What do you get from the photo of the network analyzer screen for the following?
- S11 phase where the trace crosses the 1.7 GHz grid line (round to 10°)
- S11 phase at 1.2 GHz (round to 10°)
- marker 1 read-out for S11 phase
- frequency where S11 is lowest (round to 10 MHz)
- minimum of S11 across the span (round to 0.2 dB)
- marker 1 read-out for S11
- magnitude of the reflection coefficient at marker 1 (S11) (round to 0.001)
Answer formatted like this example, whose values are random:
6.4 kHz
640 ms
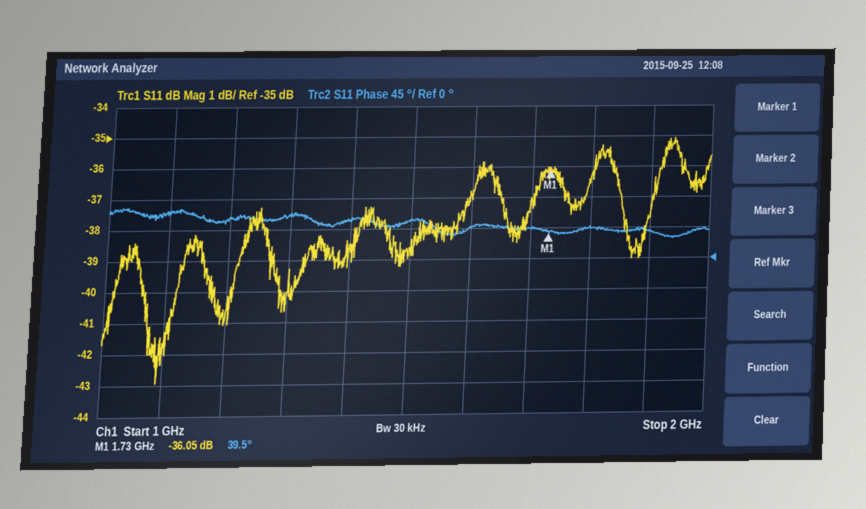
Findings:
40°
60°
39.5°
1.09 GHz
-43.0 dB
-36.05 dB
0.016
